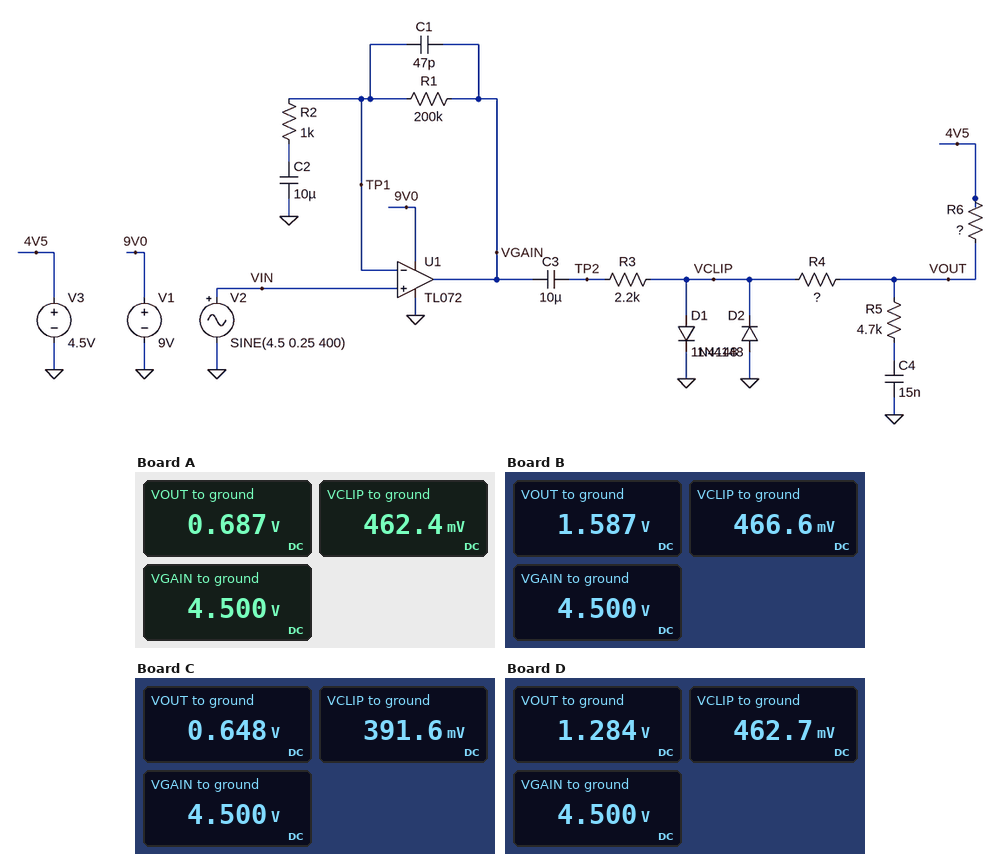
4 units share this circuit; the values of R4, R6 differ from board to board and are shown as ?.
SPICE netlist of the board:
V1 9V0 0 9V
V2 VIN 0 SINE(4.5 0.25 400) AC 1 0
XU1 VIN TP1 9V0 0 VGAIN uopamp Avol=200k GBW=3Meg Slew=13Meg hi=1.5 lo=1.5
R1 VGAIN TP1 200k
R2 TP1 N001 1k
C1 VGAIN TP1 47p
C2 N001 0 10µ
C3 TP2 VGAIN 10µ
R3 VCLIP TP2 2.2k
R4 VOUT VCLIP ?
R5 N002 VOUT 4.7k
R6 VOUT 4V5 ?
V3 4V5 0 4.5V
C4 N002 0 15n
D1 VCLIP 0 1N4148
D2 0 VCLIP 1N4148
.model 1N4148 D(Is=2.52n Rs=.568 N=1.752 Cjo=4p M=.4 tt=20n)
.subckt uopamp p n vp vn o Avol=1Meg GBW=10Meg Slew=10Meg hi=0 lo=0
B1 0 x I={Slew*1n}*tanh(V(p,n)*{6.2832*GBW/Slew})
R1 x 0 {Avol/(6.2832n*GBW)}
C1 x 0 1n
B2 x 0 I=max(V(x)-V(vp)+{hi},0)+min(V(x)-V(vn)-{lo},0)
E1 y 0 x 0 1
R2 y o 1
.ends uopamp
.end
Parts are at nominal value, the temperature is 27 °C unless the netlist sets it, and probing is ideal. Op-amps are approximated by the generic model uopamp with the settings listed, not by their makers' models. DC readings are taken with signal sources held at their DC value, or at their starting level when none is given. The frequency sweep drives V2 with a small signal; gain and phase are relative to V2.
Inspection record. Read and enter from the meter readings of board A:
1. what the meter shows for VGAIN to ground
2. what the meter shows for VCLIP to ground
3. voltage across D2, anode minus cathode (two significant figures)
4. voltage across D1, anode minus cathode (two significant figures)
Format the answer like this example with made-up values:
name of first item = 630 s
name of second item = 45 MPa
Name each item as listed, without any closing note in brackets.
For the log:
what the meter shows for VGAIN to ground = 4.500 V
what the meter shows for VCLIP to ground = 462.4 mV
voltage across D2, anode minus cathode = -460 mV
voltage across D1, anode minus cathode = 460 mV
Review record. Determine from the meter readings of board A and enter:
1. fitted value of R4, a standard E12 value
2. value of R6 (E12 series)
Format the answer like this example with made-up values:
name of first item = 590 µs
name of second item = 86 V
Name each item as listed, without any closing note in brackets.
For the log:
fitted value of R4, a standard E12 value = 3.3 kΩ
value of R6 = 56 kΩ
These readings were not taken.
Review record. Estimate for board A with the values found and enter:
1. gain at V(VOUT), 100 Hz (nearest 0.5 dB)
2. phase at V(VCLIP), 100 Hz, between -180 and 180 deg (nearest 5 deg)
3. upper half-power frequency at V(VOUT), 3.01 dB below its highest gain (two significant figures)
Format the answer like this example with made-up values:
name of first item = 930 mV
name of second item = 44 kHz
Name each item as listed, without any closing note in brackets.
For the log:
gain at V(VOUT), 100 Hz = 32.5 dB
phase at V(VCLIP), 100 Hz, between -180 and 180 deg = 10 deg
upper half-power frequency at V(VOUT), 3.01 dB below its highest gain = 2.0 kHz
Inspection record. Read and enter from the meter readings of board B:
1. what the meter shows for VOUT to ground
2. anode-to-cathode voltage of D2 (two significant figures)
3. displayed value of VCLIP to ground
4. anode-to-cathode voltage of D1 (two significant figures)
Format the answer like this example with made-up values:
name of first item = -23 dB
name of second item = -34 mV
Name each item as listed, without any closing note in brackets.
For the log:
what the meter shows for VOUT to ground = 1.587 V
anode-to-cathode voltage of D2 = -470 mV
displayed value of VCLIP to ground = 466.6 mV
anode-to-cathode voltage of D1 = 470 mV
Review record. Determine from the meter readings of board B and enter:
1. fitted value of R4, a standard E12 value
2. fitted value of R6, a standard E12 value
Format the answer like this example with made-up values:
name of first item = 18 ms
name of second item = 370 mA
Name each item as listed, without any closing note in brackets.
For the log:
fitted value of R4, a standard E12 value = 15 kΩ
fitted value of R6, a standard E12 value = 39 kΩ
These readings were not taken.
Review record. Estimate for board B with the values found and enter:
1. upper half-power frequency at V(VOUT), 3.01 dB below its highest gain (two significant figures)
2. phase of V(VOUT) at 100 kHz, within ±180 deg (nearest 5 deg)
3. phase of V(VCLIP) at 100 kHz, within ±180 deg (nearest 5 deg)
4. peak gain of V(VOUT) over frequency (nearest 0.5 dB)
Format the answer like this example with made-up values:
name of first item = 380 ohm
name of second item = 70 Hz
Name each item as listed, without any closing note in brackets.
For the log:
upper half-power frequency at V(VOUT), 3.01 dB below its highest gain = 770 Hz
phase of V(VOUT) at 100 kHz, within ±180 deg = -85 deg
phase of V(VCLIP) at 100 kHz, within ±180 deg = -85 deg
peak gain of V(VOUT) over frequency = 29.5 dB
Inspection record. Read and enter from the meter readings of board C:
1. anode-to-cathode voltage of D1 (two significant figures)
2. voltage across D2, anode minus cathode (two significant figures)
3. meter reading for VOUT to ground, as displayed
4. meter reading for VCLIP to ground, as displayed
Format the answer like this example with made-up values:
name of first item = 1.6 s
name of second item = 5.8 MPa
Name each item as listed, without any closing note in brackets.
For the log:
anode-to-cathode voltage of D1 = 390 mV
voltage across D2, anode minus cathode = -390 mV
meter reading for VOUT to ground, as displayed = 0.648 V
meter reading for VCLIP to ground, as displayed = 391.6 mV
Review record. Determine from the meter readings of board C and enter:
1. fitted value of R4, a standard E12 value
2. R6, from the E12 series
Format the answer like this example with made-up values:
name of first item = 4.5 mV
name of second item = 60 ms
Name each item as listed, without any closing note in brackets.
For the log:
fitted value of R4, a standard E12 value = 18 kΩ
R6, from the E12 series = 270 kΩ
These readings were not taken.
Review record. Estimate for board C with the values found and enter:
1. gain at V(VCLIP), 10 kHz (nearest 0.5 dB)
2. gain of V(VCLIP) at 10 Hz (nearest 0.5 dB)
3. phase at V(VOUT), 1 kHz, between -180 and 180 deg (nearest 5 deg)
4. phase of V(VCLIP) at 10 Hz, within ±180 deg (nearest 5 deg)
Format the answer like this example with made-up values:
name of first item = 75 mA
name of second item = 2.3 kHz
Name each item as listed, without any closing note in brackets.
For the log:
gain at V(VCLIP), 10 kHz = 37.0 dB
gain of V(VCLIP) at 10 Hz = 35.5 dB
phase at V(VOUT), 1 kHz, between -180 and 180 deg = -45 deg
phase of V(VCLIP) at 10 Hz, within ±180 deg = 75 deg
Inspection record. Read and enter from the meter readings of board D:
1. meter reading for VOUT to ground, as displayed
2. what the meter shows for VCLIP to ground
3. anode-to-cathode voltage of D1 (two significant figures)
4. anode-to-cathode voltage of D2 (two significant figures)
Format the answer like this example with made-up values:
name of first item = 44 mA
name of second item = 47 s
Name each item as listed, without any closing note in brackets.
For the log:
meter reading for VOUT to ground, as displayed = 1.284 V
what the meter shows for VCLIP to ground = 462.7 mV
anode-to-cathode voltage of D1 = 460 mV
anode-to-cathode voltage of D2 = -460 mV
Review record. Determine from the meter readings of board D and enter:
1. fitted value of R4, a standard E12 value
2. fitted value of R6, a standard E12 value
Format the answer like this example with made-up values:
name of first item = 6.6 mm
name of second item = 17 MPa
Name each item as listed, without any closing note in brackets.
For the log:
fitted value of R4, a standard E12 value = 12 kΩ
fitted value of R6, a standard E12 value = 47 kΩ
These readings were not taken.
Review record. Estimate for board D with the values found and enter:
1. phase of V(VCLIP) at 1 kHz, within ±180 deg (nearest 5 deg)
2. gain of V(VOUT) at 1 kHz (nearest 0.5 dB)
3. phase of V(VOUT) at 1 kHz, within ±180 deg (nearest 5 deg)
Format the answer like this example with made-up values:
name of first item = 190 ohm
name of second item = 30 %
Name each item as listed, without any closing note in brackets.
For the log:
phase of V(VCLIP) at 1 kHz, within ±180 deg = -5 deg
gain of V(VOUT) at 1 kHz = 27.5 dB
phase of V(VOUT) at 1 kHz, within ±180 deg = -35 deg
